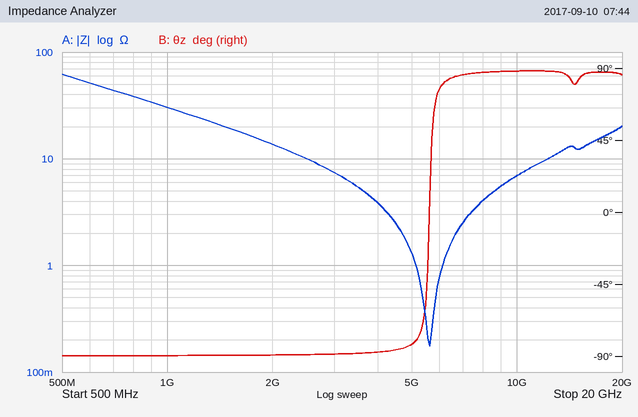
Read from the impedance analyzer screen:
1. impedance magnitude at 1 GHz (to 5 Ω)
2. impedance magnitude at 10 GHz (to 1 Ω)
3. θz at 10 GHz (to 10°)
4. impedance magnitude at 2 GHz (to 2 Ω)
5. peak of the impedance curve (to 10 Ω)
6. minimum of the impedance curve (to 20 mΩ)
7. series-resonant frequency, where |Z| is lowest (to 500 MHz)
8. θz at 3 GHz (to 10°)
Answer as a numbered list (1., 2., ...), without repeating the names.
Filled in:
1. 30 Ω
2. 7 Ω
3. 90°
4. 14 Ω
5. 60 Ω
6. 180 mΩ
7. 5.5 GHz
8. -90°
